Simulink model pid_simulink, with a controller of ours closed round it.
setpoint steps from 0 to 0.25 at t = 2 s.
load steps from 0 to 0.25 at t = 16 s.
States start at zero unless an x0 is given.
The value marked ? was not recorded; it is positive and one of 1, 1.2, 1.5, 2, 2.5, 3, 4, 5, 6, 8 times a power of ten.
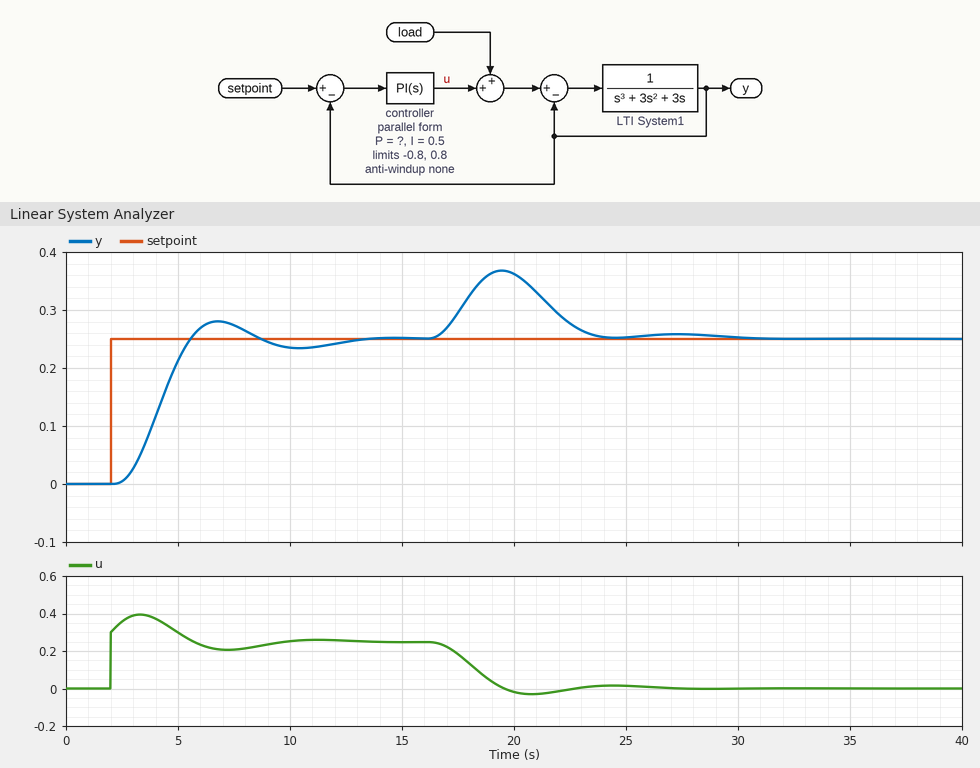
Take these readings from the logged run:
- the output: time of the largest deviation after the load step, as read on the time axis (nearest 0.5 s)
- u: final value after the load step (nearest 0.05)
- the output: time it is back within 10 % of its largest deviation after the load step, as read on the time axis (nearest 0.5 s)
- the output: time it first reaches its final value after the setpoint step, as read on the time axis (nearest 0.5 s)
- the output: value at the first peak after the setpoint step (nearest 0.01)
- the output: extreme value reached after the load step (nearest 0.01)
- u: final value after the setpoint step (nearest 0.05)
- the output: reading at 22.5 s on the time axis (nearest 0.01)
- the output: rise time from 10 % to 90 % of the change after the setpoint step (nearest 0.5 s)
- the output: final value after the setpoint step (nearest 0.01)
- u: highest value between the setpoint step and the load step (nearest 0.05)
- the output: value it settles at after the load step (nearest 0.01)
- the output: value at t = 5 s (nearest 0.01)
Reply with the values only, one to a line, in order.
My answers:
19.5 s
0.00
23.0 s
5.5 s
0.28
0.37
0.25
0.28
2.0 s
0.25
0.40
0.25
0.21
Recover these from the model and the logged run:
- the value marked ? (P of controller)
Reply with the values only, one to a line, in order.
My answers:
1.2
